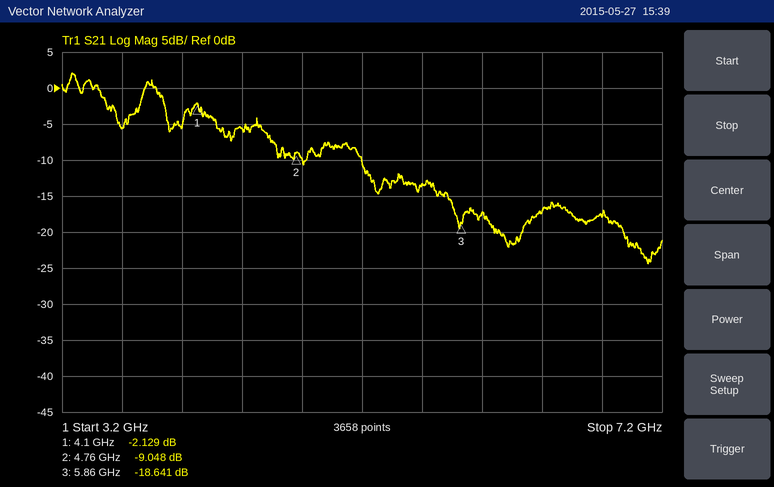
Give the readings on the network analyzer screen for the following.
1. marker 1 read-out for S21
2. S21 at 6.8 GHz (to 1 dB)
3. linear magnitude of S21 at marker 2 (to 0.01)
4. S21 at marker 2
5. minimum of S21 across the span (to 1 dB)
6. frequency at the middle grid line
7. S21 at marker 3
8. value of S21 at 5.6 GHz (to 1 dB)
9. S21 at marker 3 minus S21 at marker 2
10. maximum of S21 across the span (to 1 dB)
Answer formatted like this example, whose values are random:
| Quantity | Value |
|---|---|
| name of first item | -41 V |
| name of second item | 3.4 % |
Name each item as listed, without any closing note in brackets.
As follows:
| Quantity | Value |
|---|---|
| marker 1 read-out for S21 | -2.129 dB |
| S21 at 6.8 GHz | -18 dB |
| linear magnitude of S21 at marker 2 | 0.35 |
| S21 at marker 2 | -9.048 dB |
| minimum of S21 across the span | -24 dB |
| frequency at the middle grid line | 5.2 GHz |
| S21 at marker 3 | -18.641 dB |
| value of S21 at 5.6 GHz | -13 dB |
| S21 at marker 3 minus S21 at marker 2 | -9.593 dB |
| maximum of S21 across the span | 2 dB |
